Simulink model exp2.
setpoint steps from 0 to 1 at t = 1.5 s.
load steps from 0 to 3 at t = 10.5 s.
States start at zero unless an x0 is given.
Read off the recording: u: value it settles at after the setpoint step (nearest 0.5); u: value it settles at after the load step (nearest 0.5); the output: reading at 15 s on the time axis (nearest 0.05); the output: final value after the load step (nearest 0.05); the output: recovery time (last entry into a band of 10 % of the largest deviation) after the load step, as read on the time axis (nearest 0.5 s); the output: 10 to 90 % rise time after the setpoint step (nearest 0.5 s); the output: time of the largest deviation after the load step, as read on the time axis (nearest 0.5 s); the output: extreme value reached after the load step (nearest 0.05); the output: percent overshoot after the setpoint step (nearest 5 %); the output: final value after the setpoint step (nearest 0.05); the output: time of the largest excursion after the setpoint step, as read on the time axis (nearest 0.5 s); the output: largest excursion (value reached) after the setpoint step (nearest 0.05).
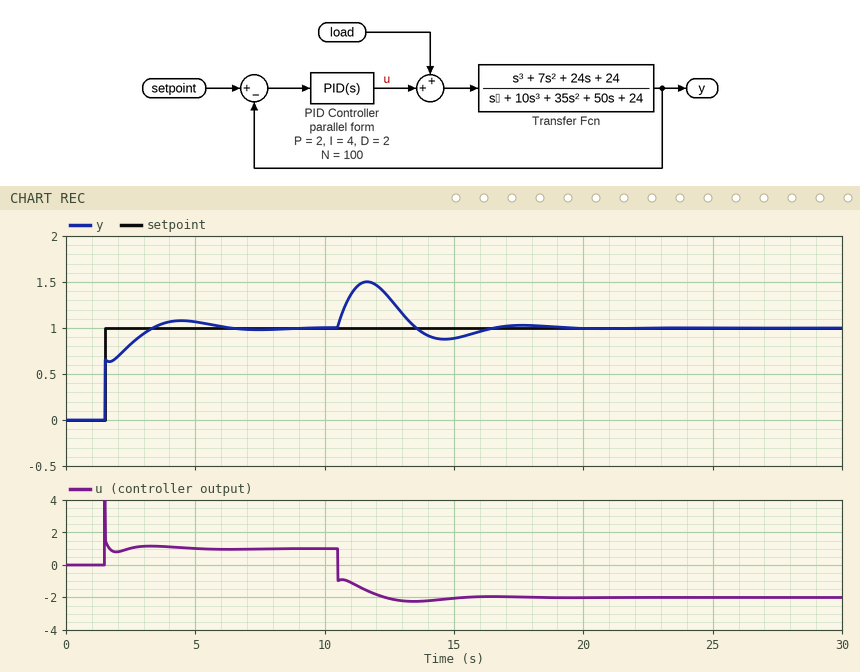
1.0
-2.0
0.90
1.00
16.0 s
1.5 s
11.5 s
1.50
10 %
1.00
4.5 s
1.10
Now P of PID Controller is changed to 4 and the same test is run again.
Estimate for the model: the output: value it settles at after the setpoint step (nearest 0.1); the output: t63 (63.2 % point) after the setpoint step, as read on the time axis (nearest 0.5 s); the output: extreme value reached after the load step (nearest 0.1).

1.0
1.5 s
1.4
